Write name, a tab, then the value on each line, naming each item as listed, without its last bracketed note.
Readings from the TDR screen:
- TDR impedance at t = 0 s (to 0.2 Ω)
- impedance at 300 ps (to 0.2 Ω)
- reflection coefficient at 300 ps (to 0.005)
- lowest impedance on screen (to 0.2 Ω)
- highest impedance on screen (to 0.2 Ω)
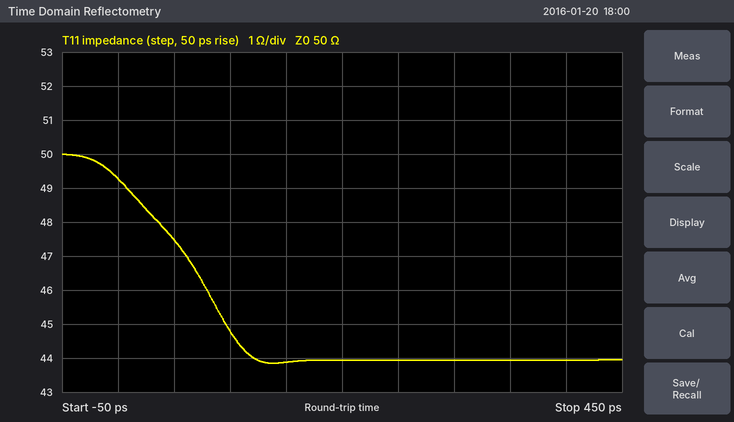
TDR impedance at t = 0 s	49.2 Ω
impedance at 300 ps	44.0 Ω
reflection coefficient at 300 ps	-0.065
lowest impedance on screen	43.8 Ω
highest impedance on screen	50.0 Ω
